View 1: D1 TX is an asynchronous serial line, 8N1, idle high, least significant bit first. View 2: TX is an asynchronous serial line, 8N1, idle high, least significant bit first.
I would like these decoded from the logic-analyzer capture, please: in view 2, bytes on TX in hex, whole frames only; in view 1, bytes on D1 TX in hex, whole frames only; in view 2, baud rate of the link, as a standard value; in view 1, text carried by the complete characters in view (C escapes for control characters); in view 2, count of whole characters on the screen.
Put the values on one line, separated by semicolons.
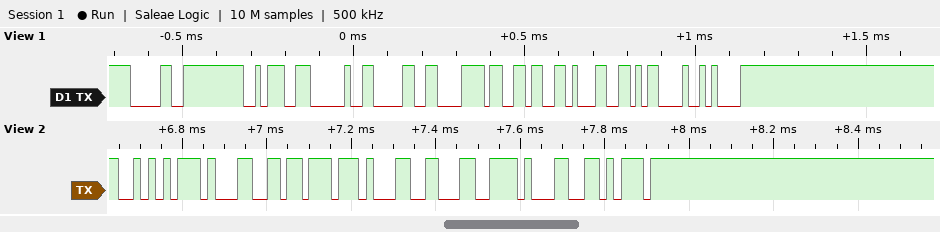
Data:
AA 31 BB 31 CC 31 DD; 0x30 0x3A 0x20 0x30 0x78 0x36 0x31 0x0D 0x0A; 57600 baud; "0: 0x61\r\n"; 7
